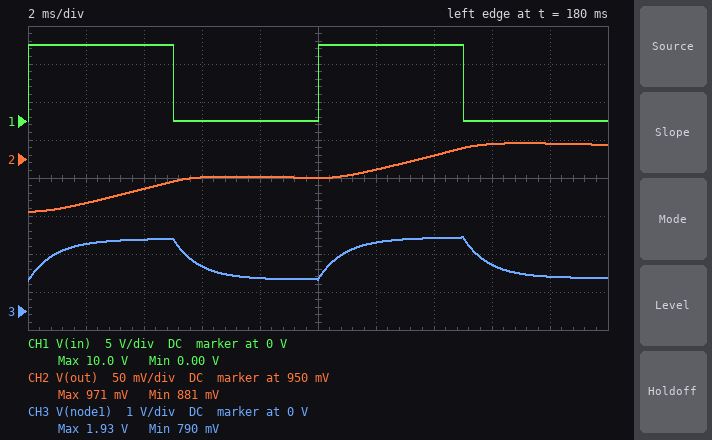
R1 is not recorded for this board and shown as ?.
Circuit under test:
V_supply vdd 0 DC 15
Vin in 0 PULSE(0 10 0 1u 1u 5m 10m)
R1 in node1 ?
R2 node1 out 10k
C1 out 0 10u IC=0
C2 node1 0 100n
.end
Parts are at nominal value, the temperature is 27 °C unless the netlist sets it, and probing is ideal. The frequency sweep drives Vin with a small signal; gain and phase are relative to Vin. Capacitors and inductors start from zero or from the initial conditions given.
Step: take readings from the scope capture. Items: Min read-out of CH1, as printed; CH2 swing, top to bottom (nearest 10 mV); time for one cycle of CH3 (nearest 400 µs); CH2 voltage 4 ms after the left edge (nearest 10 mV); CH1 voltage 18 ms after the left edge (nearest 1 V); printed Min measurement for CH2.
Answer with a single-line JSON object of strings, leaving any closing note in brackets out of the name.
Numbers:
{"Min read-out of CH1, as printed": "0.00 V", "CH2 swing, top to bottom": "90 mV", "time for one cycle of CH3": "10.0 ms", "CH2 voltage 4 ms after the left edge": "910 mV", "CH1 voltage 18 ms after the left edge": "0 V", "printed Min measurement for CH2": "881 mV"}
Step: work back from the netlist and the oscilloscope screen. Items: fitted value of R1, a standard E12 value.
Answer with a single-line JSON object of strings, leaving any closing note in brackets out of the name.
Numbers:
{"fitted value of R1, a standard E12 value": "82 kΩ"}
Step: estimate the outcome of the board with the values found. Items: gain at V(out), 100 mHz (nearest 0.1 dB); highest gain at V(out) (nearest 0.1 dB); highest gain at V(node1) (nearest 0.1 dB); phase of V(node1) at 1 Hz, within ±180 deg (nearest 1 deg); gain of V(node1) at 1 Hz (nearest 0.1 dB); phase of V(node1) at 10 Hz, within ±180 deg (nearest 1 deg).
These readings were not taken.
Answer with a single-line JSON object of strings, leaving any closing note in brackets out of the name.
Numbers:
{"gain at V(out), 100 mHz": "-1.3 dB", "highest gain at V(out)": "0 dB", "highest gain at V(node1)": "0 dB", "phase of V(node1) at 1 Hz, within ±180 deg": "-48 deg", "gain of V(node1) at 1 Hz": "-14.0 dB", "phase of V(node1) at 10 Hz, within ±180 deg": "-11 deg"}
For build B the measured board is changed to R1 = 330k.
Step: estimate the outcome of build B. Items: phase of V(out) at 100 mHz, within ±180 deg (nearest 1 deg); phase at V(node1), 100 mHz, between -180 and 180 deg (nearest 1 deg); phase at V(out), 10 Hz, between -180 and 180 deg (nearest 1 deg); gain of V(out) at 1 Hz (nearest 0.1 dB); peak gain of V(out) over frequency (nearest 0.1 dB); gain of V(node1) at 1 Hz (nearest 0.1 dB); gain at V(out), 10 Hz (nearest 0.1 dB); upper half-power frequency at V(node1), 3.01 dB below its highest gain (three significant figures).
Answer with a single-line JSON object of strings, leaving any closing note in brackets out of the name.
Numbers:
{"phase of V(out) at 100 mHz, within ±180 deg": "-65 deg", "phase at V(node1), 100 mHz, between -180 and 180 deg": "-62 deg", "phase at V(out), 10 Hz, between -180 and 180 deg": "-93 deg", "gain of V(out) at 1 Hz": "-26.7 dB", "peak gain of V(out) over frequency": "0 dB", "gain of V(node1) at 1 Hz": "-25.2 dB", "gain at V(out), 10 Hz": "-46.7 dB", "upper half-power frequency at V(node1), 3.01 dB below its highest gain": "46.4 mHz"}
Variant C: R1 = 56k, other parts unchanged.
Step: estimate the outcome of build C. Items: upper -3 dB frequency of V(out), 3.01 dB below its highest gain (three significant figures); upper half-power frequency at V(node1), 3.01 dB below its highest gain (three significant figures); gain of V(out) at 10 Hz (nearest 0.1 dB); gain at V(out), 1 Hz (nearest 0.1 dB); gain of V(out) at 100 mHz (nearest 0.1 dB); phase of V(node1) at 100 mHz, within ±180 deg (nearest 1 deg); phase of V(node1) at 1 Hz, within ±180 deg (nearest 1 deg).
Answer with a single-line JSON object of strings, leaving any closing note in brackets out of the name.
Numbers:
{"upper -3 dB frequency of V(out), 3.01 dB below its highest gain": "239 mHz", "upper half-power frequency at V(node1), 3.01 dB below its highest gain": "245 mHz", "gain of V(out) at 10 Hz": "-32.4 dB", "gain at V(out), 1 Hz": "-12.7 dB", "gain of V(out) at 100 mHz": "-0.7 dB", "phase of V(node1) at 100 mHz, within ±180 deg": "-19 deg", "phase of V(node1) at 1 Hz, within ±180 deg": "-45 deg"}
